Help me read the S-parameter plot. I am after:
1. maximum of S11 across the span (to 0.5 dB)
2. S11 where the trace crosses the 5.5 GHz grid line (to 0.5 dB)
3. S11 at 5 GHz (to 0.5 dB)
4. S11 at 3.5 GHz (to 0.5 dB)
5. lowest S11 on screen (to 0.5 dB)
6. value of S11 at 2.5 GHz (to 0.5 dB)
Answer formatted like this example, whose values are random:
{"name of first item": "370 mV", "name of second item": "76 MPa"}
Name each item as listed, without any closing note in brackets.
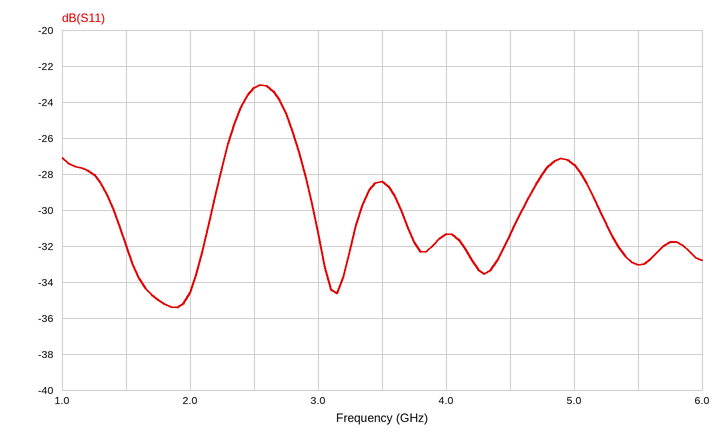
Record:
{"maximum of S11 across the span": "-23.0 dB", "S11 where the trace crosses the 5.5 GHz grid line": "-33.0 dB", "S11 at 5 GHz": "-27.5 dB", "S11 at 3.5 GHz": "-28.5 dB", "lowest S11 on screen": "-35.5 dB", "value of S11 at 2.5 GHz": "-23.0 dB"}
